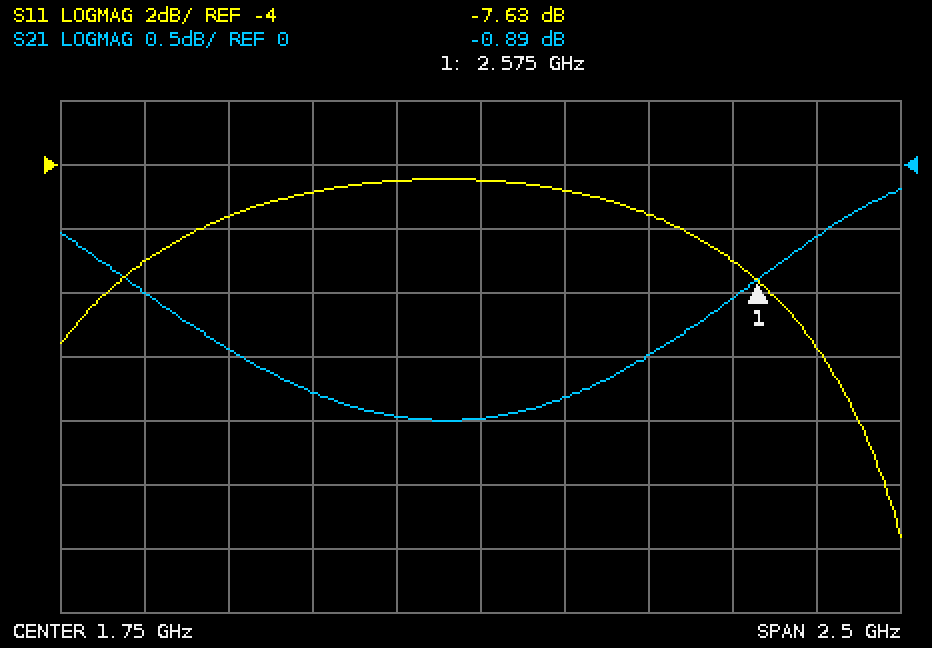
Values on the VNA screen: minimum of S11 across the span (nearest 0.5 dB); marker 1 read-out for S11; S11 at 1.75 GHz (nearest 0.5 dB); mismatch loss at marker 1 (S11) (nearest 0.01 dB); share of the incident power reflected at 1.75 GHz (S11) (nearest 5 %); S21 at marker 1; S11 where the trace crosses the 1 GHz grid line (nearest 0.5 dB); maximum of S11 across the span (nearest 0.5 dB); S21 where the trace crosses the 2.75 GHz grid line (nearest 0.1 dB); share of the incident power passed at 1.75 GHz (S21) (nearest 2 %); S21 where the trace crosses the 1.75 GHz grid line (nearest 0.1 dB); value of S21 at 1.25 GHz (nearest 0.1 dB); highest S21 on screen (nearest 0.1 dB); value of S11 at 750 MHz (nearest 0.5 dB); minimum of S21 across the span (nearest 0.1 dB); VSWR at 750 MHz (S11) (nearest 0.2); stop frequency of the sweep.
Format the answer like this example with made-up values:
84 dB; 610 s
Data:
-15.5 dB; -7.63 dB; -4.5 dB; 0.82 dB; 35 %; -0.89 dB; -5.5 dB; -4.5 dB; -0.6 dB; 64 %; -2.0 dB; -1.8 dB; -0.2 dB; -7.0 dB; -2.0 dB; 2.6; 3 GHz
